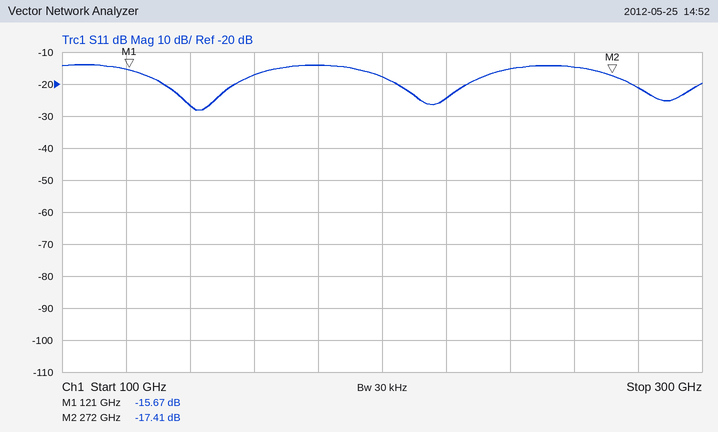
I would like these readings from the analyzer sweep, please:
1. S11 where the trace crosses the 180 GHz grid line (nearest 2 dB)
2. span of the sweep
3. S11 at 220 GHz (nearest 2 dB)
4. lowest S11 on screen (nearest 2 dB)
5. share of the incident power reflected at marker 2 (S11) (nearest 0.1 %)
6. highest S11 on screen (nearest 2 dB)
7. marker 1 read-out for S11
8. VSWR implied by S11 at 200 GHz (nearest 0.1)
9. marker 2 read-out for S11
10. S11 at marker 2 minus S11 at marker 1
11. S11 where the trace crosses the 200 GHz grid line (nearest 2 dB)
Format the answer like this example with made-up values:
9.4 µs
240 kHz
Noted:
-14 dB
200 GHz
-24 dB
-28 dB
1.8 %
-14 dB
-15.67 dB
1.3
-17.41 dB
-1.74 dB
-18 dB
